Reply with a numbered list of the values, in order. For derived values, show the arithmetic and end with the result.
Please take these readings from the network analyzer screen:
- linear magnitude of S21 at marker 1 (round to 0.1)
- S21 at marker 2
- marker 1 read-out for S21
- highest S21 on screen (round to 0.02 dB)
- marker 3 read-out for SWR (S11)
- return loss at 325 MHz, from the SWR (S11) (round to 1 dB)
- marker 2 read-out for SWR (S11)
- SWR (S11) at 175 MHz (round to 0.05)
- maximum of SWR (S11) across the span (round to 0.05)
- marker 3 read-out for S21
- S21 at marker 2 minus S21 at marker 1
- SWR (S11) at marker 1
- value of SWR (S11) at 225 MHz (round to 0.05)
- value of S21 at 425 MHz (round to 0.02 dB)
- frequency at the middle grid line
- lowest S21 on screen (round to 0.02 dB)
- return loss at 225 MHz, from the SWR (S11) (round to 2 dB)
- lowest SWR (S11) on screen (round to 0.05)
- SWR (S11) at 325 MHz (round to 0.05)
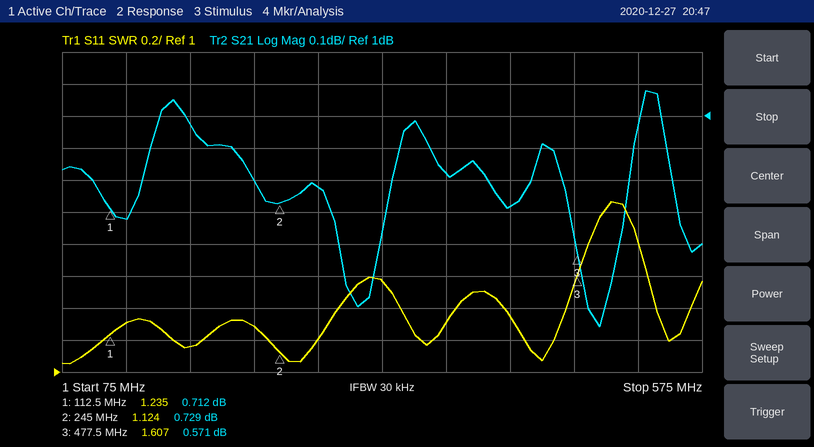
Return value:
1. 10^(0.712/20) ≈ 1.1
2. 0.729 dB
3. 0.712 dB
4. 1.08 dB
5. 1.607
6. −20 log10((1.55 − 1)/(1.55 + 1)) ≈ 13 dB
7. 1.124
8. 1.15
9. 2.05
10. 0.571 dB
11. 0.729 − (0.712) = 0.017 dB
12. 1.235
13. 1.30
14. 0.72 dB
15. 325 MHz
16. 0.34 dB
17. −20 log10((1.3 − 1)/(1.3 + 1)) ≈ 18 dB
18. 1.05
19. 1.55
